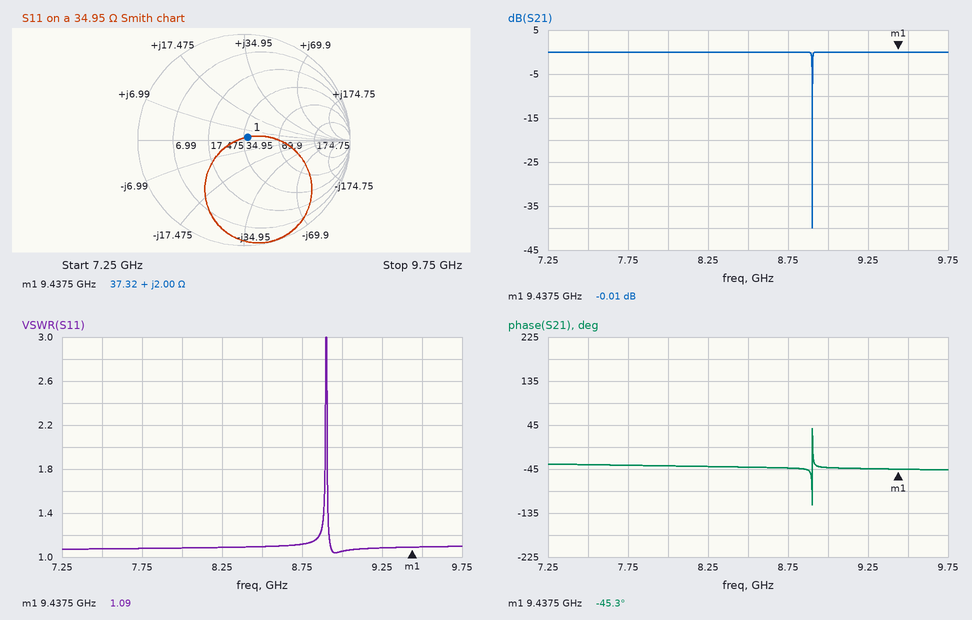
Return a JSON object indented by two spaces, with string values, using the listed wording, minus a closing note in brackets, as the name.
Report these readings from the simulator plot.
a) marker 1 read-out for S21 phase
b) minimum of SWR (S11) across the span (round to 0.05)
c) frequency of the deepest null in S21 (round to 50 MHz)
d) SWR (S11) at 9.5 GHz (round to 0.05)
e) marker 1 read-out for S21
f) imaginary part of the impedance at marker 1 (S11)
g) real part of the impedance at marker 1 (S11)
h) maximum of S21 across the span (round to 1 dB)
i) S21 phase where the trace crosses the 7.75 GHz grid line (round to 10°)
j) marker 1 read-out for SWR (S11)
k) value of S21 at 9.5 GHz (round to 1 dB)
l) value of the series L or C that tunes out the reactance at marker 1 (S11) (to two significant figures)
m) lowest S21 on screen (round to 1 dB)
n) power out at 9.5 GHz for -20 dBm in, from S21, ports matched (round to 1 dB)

{
  "marker 1 read-out for S21 phase": "-45.3°",
  "minimum of SWR (S11) across the span": "1.05",
  "frequency of the deepest null in S21": "8.90 GHz",
  "SWR (S11) at 9.5 GHz": "1.10",
  "marker 1 read-out for S21": "-0.01 dB",
  "imaginary part of the impedance at marker 1": "+2.00 Ω",
  "real part of the impedance at marker 1": "37.32 Ω",
  "maximum of S21 across the span": "0 dB",
  "S21 phase where the trace crosses the 7.75 GHz grid line": "-40°",
  "marker 1 read-out for SWR": "1.09",
  "value of S21 at 9.5 GHz": "0 dB",
  "value of the series L or C that tunes out the reactance at marker 1 (S11)": "8.4 pF",
  "lowest S21 on screen": "-40 dB",
  "power out at 9.5 GHz for -20 dBm in, from S21, ports matched": "-20 dBm"
}
